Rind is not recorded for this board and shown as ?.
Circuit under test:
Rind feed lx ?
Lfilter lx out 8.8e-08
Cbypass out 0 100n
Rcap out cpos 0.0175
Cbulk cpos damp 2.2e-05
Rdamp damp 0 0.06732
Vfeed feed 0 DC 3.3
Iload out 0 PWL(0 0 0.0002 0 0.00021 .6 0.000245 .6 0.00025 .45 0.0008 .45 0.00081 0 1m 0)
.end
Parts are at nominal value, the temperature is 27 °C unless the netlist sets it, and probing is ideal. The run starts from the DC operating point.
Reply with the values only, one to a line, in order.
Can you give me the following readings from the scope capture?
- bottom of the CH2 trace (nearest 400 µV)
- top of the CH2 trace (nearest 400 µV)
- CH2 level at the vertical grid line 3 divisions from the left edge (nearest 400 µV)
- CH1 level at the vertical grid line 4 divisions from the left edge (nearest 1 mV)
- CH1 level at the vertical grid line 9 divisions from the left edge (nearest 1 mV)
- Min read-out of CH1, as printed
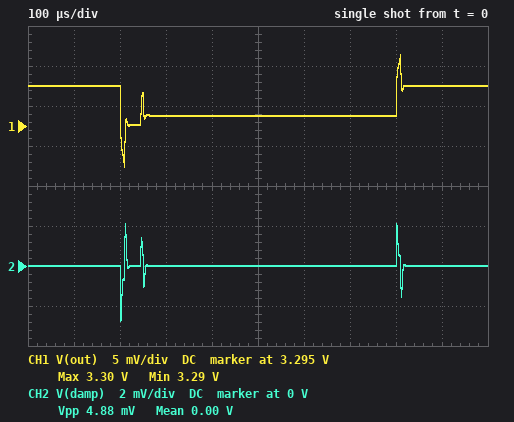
-2.8 mV
2.0 mV
0 V
3.296 V
3.300 V
3.29 V
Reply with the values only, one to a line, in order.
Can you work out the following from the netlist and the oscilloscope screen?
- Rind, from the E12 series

8.2 mΩ
